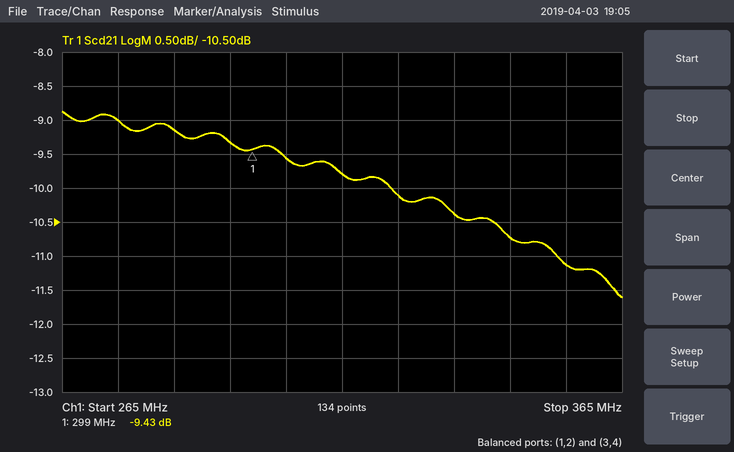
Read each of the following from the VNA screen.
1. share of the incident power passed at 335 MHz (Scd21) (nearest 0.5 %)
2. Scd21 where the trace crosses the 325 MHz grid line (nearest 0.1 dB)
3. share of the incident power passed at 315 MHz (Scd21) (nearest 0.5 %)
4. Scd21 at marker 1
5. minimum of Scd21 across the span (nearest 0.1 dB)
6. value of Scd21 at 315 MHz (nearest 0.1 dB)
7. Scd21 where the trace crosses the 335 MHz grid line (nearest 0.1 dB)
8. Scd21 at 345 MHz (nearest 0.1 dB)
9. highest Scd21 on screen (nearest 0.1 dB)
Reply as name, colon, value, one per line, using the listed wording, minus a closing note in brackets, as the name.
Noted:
share of the incident power passed at 335 MHz (Scd21): 9.0 %
Scd21 where the trace crosses the 325 MHz grid line: -10.1 dB
share of the incident power passed at 315 MHz (Scd21): 10.5 %
Scd21 at marker 1: -9.43 dB
minimum of Scd21 across the span: -11.6 dB
value of Scd21 at 315 MHz: -9.8 dB
Scd21 where the trace crosses the 335 MHz grid line: -10.4 dB
Scd21 at 345 MHz: -10.7 dB
highest Scd21 on screen: -8.9 dB
